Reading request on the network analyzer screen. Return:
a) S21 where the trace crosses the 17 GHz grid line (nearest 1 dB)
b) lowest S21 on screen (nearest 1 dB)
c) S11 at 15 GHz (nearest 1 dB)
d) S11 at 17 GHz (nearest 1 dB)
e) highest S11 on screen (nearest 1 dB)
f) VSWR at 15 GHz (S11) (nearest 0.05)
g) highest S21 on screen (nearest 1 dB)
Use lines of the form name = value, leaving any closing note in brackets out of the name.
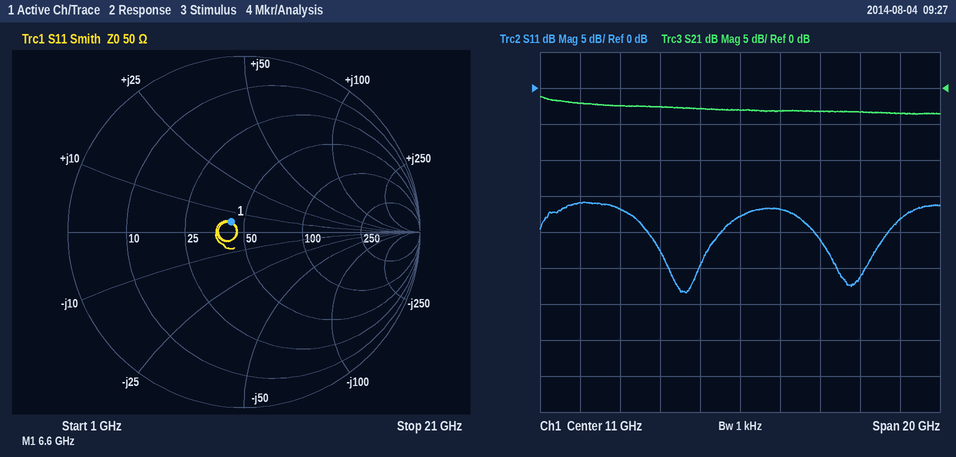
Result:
S21 where the trace crosses the 17 GHz grid line = -3 dB
lowest S21 on screen = -4 dB
S11 at 15 GHz = -21 dB
S11 at 17 GHz = -26 dB
highest S11 on screen = -16 dB
VSWR at 15 GHz (S11) = 1.20
highest S21 on screen = -1 dB
